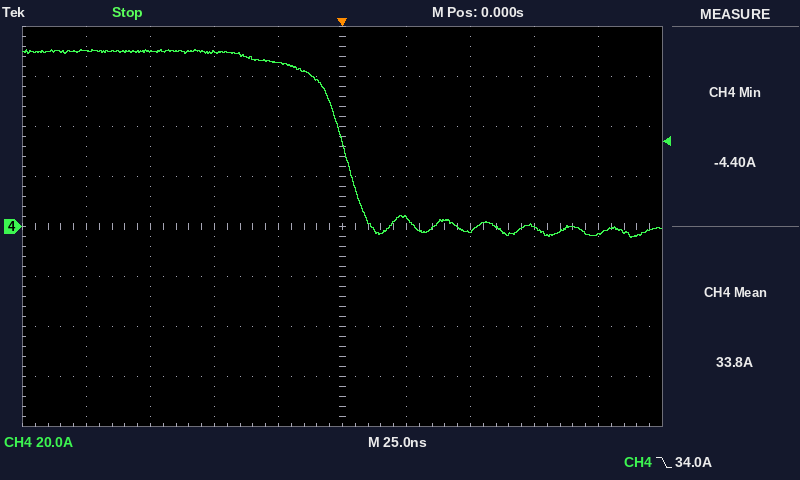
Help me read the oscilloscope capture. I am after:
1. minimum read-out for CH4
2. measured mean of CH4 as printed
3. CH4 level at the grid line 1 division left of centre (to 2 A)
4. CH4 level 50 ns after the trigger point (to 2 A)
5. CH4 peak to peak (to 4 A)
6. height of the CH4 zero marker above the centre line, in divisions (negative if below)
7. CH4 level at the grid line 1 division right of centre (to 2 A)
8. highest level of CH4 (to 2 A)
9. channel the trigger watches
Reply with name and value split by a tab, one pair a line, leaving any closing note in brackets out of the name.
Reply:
minimum read-out for CH4	-4.40 A
measured mean of CH4 as printed	33.8 A
CH4 level at the grid line 1 division left of centre	66 A
CH4 level 50 ns after the trigger point	-2 A
CH4 peak to peak	76 A
height of the CH4 zero marker above the centre line, in divisions	0.0 div
CH4 level at the grid line 1 division right of centre	4 A
highest level of CH4	70 A
channel the trigger watches	CH4
